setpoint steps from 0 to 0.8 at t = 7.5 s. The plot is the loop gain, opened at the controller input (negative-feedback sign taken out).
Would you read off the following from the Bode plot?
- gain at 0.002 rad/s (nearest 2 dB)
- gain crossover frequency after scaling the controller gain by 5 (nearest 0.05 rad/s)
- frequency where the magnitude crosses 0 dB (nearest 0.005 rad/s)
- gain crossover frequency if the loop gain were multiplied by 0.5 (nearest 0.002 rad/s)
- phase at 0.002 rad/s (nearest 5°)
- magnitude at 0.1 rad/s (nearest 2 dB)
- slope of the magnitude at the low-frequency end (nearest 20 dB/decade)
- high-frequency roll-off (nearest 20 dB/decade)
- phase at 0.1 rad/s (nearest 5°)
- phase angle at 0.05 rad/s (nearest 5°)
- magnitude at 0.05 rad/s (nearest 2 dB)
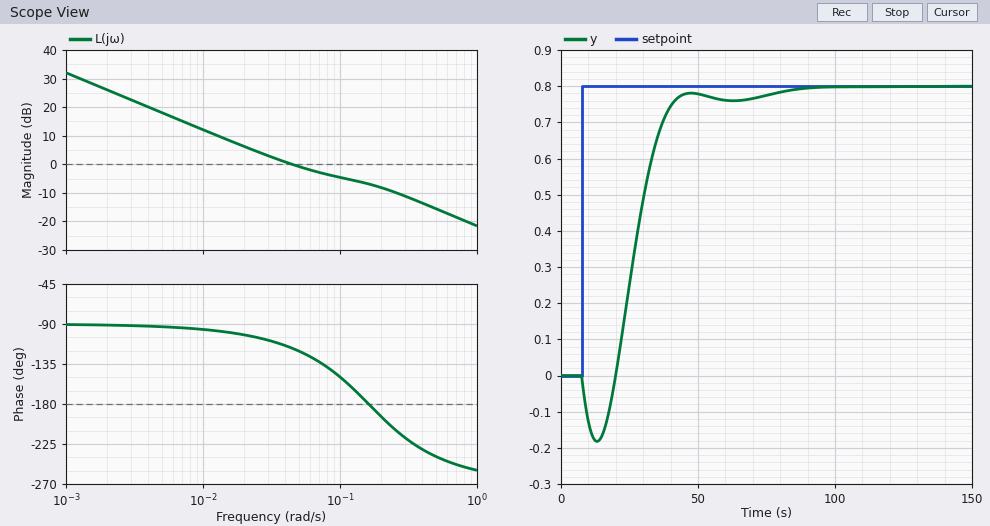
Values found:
26 dB
0.40 rad/s
0.045 rad/s
0.020 rad/s
-90°
-4 dB
-20 dB/decade
-20 dB/decade
-150°
-120°
0 dB
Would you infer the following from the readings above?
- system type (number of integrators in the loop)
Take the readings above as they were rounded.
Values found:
1
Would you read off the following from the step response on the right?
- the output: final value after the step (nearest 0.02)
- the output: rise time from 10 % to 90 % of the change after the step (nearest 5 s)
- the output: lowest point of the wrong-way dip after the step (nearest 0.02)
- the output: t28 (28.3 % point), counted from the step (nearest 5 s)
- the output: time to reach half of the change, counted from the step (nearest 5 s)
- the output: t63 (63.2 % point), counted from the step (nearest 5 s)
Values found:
0.80
15 s
-0.18
15 s
20 s
25 s
